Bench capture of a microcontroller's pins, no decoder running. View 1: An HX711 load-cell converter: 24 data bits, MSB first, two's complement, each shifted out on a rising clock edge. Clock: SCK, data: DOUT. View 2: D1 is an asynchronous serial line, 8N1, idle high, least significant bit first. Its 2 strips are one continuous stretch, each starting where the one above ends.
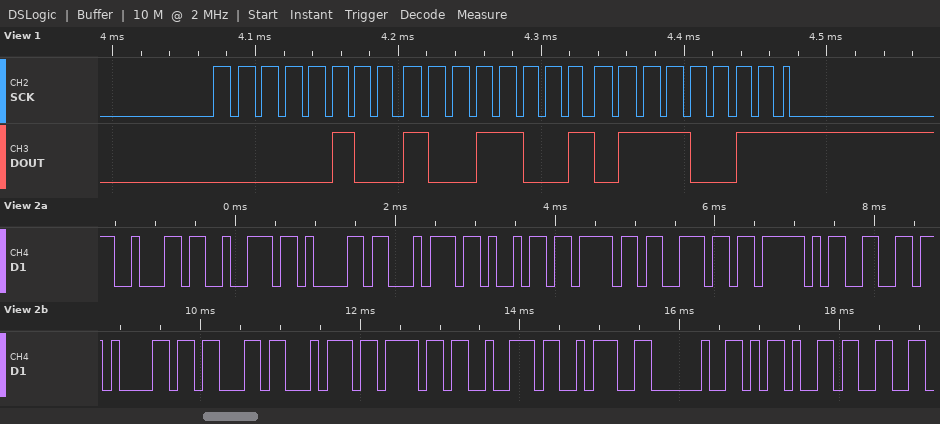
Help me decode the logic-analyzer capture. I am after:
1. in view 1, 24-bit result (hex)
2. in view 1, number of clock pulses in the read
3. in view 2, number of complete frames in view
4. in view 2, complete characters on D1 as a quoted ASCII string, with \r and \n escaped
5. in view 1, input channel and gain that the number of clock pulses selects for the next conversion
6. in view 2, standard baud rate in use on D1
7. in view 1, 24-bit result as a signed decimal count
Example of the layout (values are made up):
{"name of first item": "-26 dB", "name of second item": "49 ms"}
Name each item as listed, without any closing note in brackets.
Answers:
{"in view 1, 24-bit result": "0x049973", "in view 1, number of clock pulses in the read": "25", "in view 2, number of complete frames in view": "18", "in view 2, complete characters on D1 as a quoted ASCII string, with \\r and \\n escaped": "\"bration_factor: -3\"", "in view 1, input channel and gain that the number of clock pulses selects for the next conversion": "channel A, gain 128", "in view 2, standard baud rate in use on D1": "9600 baud", "in view 1, 24-bit result as a signed decimal count": "301427"}
